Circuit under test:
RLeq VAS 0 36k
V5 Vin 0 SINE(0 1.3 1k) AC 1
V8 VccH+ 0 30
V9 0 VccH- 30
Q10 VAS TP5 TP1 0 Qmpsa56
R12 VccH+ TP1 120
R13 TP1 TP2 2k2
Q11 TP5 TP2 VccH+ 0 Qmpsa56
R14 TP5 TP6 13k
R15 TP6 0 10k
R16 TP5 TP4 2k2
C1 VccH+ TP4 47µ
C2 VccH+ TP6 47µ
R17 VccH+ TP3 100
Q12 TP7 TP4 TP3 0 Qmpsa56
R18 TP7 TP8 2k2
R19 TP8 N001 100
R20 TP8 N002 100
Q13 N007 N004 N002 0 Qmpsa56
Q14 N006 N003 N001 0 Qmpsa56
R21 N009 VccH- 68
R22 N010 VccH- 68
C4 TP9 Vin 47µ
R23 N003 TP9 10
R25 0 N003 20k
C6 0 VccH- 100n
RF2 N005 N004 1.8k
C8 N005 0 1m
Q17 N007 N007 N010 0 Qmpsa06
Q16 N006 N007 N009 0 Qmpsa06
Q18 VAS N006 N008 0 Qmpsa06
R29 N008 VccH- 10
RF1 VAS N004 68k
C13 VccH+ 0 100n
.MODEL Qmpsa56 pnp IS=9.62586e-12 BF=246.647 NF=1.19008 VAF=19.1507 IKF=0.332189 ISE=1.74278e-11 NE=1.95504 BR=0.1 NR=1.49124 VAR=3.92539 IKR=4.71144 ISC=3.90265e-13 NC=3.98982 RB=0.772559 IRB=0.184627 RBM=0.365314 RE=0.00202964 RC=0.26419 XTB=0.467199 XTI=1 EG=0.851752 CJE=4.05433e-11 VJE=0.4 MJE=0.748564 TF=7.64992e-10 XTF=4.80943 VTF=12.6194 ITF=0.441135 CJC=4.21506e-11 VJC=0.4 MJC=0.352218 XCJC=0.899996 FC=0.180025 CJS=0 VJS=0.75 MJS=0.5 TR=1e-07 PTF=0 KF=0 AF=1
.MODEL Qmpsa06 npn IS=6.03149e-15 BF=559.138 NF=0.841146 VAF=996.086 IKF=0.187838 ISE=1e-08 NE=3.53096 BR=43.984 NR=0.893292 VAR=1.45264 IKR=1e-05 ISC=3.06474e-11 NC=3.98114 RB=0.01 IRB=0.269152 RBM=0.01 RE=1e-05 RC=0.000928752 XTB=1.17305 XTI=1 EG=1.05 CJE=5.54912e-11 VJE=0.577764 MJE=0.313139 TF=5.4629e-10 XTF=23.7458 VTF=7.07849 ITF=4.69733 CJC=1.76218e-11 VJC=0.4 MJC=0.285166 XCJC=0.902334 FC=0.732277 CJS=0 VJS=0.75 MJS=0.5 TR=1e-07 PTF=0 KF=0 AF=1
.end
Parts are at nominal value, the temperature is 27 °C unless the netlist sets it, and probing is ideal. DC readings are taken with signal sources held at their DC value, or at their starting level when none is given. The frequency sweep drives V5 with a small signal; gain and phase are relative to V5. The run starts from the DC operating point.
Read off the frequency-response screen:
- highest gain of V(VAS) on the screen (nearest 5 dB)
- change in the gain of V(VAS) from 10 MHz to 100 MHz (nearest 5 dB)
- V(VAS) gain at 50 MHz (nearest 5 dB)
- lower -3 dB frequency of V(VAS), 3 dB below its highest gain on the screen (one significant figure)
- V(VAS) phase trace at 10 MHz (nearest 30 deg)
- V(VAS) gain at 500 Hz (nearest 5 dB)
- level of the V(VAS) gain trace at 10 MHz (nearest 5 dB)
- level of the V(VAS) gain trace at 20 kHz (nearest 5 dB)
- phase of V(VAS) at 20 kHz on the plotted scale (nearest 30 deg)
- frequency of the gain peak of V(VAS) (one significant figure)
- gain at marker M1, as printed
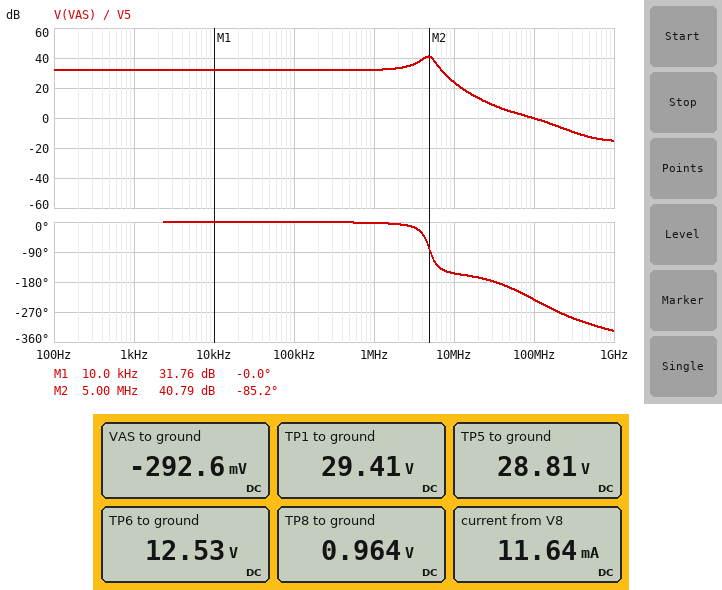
40 dB
-25 dB
5 dB
4 MHz
-150 deg
30 dB
25 dB
30 dB
0 deg
5 MHz
31.76 dB
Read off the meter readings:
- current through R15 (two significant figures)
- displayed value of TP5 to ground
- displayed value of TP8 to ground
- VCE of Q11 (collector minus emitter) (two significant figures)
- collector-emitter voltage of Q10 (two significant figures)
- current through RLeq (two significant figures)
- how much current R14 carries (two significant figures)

1.3 mA
28.81 V
0.964 V
-1.2 V
-30 V
8.1 µA
1.3 mA
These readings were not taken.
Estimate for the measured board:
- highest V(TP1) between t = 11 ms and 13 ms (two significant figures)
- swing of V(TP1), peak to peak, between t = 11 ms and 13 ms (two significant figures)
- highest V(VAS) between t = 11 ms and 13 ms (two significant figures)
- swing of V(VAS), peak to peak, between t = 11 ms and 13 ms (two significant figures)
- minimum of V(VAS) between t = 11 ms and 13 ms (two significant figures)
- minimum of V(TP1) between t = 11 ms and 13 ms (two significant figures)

30 V
290 mV
30 V
60 V
-30 V
29 V
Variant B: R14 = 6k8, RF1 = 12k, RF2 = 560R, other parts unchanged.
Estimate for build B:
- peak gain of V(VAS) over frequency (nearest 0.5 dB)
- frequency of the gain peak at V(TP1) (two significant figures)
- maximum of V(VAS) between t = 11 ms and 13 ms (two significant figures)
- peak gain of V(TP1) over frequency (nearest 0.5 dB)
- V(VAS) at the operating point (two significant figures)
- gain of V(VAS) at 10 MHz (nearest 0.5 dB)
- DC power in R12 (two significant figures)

36.5 dB
9.4 MHz
29 V
10.5 dB
48 mV
35.0 dB
3.1 mW
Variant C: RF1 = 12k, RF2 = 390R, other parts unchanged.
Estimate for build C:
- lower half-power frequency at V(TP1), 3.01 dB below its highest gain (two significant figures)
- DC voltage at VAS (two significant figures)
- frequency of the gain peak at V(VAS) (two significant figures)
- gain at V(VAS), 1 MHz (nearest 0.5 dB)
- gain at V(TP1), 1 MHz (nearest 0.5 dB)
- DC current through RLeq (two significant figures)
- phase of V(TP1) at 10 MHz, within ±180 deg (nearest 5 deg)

6.2 MHz
47 mV
7.6 MHz
30.0 dB
-18.5 dB
1.3 µA
-50 deg
